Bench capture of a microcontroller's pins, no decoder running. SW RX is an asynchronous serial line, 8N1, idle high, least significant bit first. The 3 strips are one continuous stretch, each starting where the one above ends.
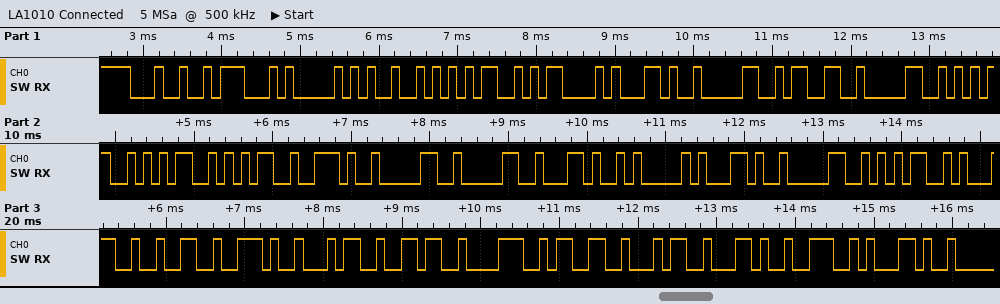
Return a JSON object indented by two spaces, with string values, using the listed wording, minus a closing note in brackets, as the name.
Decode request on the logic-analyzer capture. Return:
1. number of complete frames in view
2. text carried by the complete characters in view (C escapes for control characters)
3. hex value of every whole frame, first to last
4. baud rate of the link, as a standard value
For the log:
{
  "number of complete frames in view": "32",
  "text carried by the complete characters in view": "\"$GPRMC,030555.00,A,0512.46834,N,\"",
  "hex value of every whole frame, first to last": "24 47 50 52 4D 43 2C 30 33 30 35 35 35 2E 30 30 2C 41 2C 30 35 31 32 2E 34 36 38 33 34 2C 4E 2C",
  "baud rate of the link, as a standard value": "9600 baud"
}
